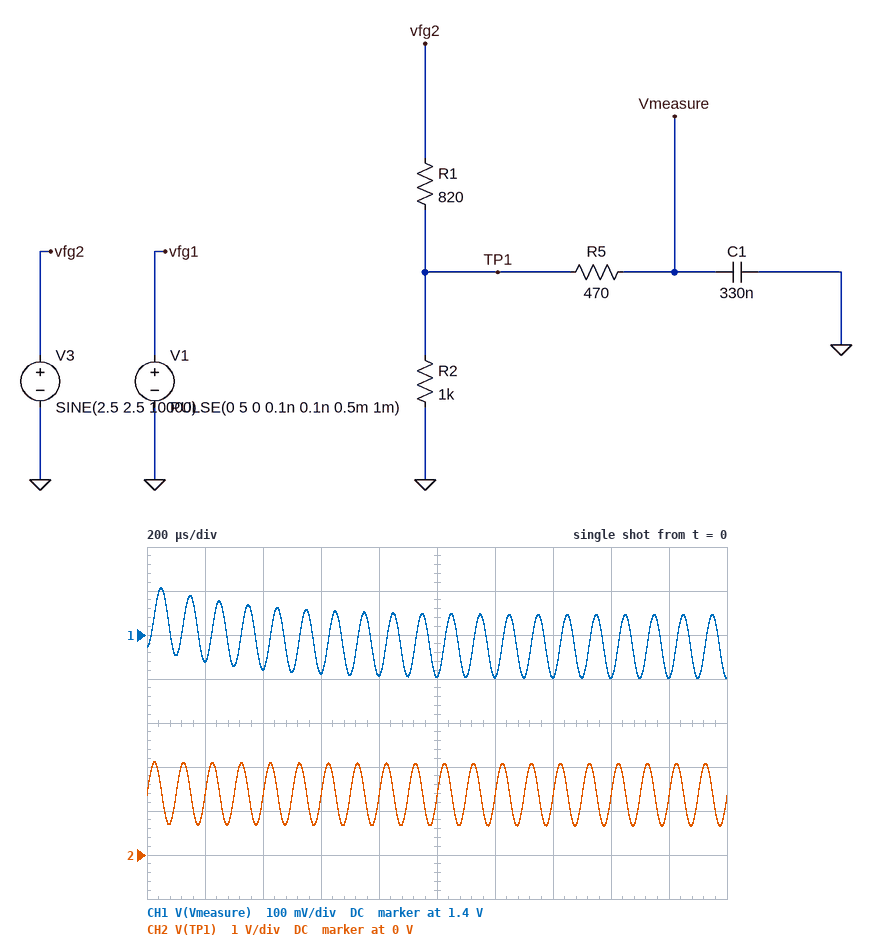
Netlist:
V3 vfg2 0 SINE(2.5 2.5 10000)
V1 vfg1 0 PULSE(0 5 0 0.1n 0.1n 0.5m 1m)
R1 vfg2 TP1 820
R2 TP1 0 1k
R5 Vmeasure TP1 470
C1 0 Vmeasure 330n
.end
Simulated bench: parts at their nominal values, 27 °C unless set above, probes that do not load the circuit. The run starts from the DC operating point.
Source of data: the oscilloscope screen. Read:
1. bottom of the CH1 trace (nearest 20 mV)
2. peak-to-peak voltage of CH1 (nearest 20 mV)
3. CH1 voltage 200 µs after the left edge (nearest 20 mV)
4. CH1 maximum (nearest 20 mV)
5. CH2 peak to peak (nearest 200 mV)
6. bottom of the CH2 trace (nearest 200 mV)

1.30 V
200 mV
1.34 V
1.50 V
1.4 V
600 mV
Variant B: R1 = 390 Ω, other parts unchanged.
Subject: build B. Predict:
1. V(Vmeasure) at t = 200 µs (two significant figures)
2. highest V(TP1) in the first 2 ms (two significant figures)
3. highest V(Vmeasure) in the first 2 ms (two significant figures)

1.7 V
3.0 V
2.0 V
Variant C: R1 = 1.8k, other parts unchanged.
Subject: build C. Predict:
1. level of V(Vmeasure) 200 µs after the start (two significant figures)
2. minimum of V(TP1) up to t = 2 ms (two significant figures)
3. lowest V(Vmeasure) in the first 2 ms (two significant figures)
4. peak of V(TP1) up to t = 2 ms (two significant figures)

880 mV
510 mV
850 mV
1.3 V
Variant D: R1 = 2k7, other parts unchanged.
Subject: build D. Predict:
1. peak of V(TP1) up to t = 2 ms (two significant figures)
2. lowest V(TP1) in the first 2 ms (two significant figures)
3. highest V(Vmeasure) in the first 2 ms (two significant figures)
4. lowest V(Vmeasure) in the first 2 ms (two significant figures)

960 mV
410 mV
730 mV
650 mV
